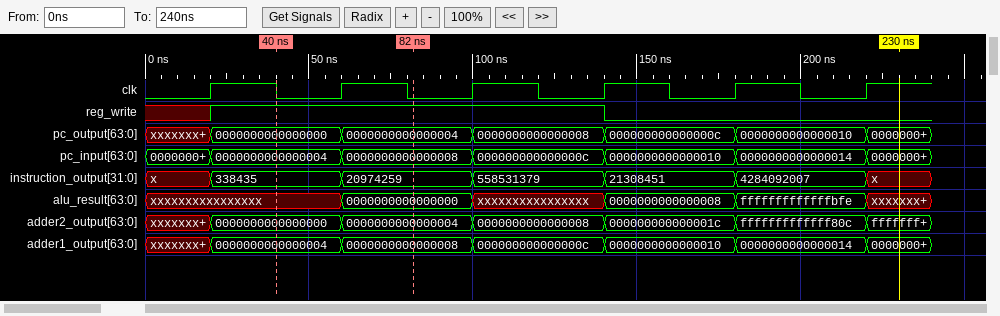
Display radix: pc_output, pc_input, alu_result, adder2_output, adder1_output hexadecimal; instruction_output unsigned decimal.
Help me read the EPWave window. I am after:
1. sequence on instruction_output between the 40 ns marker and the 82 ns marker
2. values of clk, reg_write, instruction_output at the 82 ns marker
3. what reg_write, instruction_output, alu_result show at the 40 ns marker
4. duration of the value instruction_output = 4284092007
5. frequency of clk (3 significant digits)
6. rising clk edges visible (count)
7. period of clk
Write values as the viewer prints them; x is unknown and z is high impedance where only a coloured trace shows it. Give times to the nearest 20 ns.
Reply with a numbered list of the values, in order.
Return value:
1. 338435, 20974259
2. clk=0, reg_write=1, instruction_output=20974259
3. reg_write=1, instruction_output=338435, alu_result=xxxxxxxxxxxxxxxx
4. 40 ns
5. 25.0 MHz
6. 6
7. 40 ns
